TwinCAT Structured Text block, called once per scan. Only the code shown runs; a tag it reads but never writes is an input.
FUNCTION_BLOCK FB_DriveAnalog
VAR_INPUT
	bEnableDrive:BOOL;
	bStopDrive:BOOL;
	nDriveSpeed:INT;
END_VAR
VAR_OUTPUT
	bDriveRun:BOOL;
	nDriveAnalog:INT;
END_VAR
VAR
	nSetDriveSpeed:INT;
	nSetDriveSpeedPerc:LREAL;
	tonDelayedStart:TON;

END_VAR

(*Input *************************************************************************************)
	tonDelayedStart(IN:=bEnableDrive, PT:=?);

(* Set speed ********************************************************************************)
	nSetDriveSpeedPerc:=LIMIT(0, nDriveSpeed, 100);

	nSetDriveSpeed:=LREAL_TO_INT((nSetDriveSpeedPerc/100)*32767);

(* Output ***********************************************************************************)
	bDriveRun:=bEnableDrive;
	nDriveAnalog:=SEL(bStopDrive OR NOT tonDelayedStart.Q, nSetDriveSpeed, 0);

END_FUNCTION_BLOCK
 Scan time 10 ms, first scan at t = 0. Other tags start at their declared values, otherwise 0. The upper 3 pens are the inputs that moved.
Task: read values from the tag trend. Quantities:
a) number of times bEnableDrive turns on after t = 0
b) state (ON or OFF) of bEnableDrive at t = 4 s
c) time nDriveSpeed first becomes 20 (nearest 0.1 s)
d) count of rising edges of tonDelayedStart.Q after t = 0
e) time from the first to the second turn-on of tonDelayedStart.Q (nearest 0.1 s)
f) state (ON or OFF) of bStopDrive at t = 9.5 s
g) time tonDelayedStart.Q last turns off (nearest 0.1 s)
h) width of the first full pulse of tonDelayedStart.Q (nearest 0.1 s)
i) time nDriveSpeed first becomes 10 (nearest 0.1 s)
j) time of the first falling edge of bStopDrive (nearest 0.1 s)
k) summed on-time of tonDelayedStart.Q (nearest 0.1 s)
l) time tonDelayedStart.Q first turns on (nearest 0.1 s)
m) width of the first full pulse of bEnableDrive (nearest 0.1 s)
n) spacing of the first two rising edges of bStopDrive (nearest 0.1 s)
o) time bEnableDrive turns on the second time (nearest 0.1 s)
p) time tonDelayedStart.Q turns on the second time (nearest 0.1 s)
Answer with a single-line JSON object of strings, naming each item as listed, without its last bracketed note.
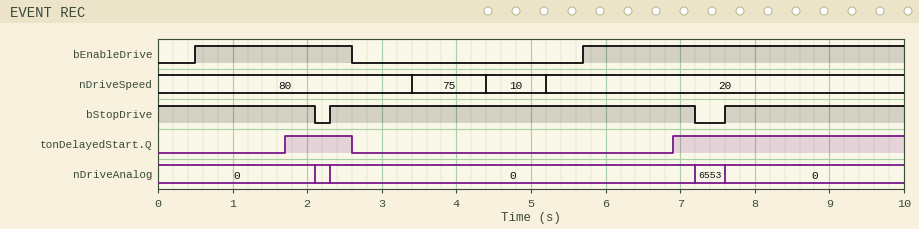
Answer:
{"number of times bEnableDrive turns on after t = 0": "2", "state (ON or OFF) of bEnableDrive at t = 4 s": "OFF", "time nDriveSpeed first becomes 20": "5.2 s", "count of rising edges of tonDelayedStart.Q after t = 0": "2", "time from the first to the second turn-on of tonDelayedStart.Q": "5.2 s", "state (ON or OFF) of bStopDrive at t = 9.5 s": "ON", "time tonDelayedStart.Q last turns off": "2.6 s", "width of the first full pulse of tonDelayedStart.Q": "0.9 s", "time nDriveSpeed first becomes 10": "4.4 s", "time of the first falling edge of bStopDrive": "2.1 s", "summed on-time of tonDelayedStart.Q": "4.0 s", "time tonDelayedStart.Q first turns on": "1.7 s", "width of the first full pulse of bEnableDrive": "2.1 s", "spacing of the first two rising edges of bStopDrive": "5.3 s", "time bEnableDrive turns on the second time": "5.7 s", "time tonDelayedStart.Q turns on the second time": "6.9 s"}
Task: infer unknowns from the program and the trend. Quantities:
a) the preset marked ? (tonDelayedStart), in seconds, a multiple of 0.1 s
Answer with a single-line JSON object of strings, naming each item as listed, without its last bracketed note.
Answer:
{"the preset marked ? (tonDelayedStart), in seconds, a multiple of 0.1 s": "1.2 s"}
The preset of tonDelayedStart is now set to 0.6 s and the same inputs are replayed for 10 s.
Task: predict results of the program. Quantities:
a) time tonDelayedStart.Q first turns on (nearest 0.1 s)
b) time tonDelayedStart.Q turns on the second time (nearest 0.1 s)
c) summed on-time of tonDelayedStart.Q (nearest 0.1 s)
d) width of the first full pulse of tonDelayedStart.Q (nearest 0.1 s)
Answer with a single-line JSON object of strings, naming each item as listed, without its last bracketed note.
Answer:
{"time tonDelayedStart.Q first turns on": "1.1 s", "time tonDelayedStart.Q turns on the second time": "6.3 s", "summed on-time of tonDelayedStart.Q": "5.2 s", "width of the first full pulse of tonDelayedStart.Q": "1.5 s"}
